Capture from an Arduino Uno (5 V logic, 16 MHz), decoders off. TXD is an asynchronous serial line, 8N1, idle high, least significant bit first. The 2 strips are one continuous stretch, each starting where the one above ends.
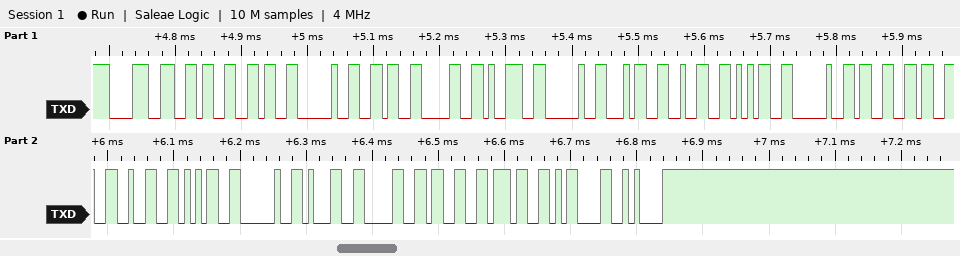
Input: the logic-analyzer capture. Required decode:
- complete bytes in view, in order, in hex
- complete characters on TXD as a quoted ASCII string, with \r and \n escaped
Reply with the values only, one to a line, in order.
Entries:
38 36 36 20 36 30 39 20 34 32 35 20 33 33 32 35 20 31 30 33 37 0D 0A
"866 609 425 3325 1037\r\n"
